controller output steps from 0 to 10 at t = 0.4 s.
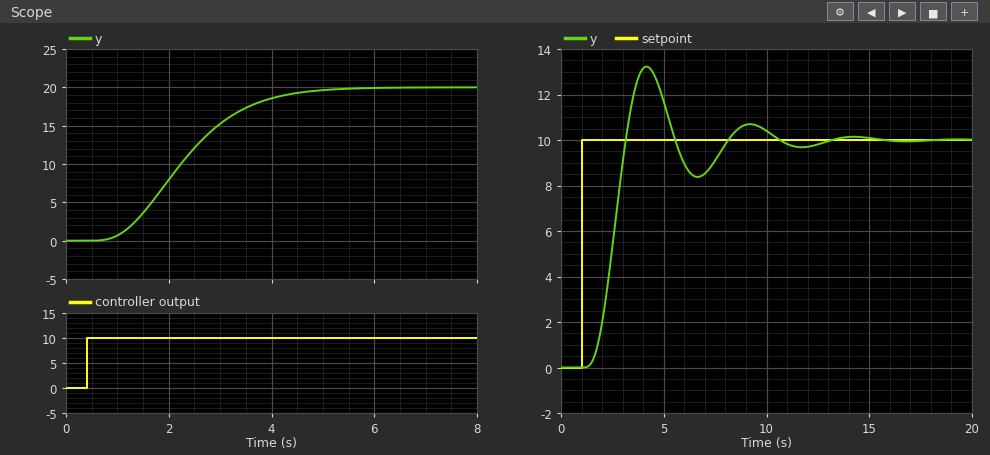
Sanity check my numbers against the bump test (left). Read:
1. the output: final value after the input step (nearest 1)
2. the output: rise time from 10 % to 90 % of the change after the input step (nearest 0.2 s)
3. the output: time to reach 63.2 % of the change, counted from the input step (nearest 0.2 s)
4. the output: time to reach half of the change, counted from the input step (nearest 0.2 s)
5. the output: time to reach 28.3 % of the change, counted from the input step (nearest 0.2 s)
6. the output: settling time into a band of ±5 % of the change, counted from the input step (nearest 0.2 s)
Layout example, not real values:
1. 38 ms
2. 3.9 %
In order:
1. 20
2. 2.4 s
3. 2.2 s
4. 1.8 s
5. 1.4 s
6. 3.8 s
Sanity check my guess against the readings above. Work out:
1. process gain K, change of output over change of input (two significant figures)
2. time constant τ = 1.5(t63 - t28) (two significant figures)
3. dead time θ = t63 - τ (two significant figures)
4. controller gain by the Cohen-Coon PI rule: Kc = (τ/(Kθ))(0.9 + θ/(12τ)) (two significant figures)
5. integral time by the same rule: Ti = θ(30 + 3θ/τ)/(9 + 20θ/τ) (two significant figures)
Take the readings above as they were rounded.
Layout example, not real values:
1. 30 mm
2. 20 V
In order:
1. 2.0
2. 1.2 s
3. 1.0 s
4. 0.58
5. 1.3 s
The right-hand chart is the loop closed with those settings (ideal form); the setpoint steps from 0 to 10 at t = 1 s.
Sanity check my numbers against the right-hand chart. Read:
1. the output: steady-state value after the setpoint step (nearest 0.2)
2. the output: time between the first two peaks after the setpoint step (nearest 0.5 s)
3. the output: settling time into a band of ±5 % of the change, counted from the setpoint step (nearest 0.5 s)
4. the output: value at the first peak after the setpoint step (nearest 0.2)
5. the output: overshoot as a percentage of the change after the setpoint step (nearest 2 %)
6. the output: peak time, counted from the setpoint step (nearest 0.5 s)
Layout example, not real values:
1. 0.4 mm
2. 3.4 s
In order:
1. 10.0
2. 5.0 s
3. 9.0 s
4. 13.2
5. 32 %
6. 3.0 s
